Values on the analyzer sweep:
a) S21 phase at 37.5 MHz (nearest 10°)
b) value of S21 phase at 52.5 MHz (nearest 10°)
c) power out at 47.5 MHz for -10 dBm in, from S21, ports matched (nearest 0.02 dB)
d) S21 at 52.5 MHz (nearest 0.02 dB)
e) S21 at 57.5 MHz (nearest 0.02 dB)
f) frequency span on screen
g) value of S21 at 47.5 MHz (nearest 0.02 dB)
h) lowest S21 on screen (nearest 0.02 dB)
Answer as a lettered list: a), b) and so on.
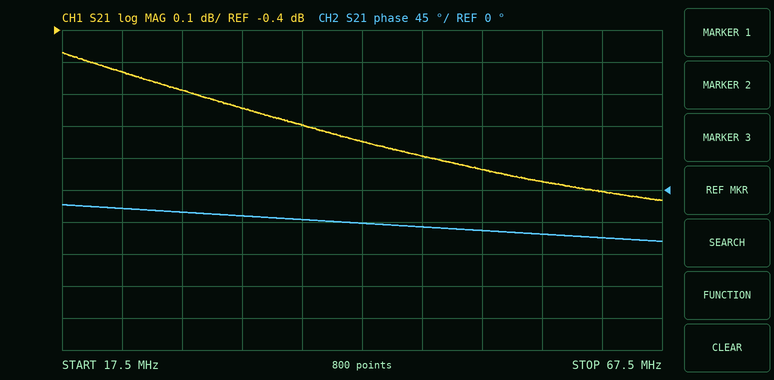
a) -40°
b) -60°
c) -10.80 dBm
d) -0.84 dB
e) -0.88 dB
f) 50 MHz
g) -0.80 dB
h) -0.94 dB
